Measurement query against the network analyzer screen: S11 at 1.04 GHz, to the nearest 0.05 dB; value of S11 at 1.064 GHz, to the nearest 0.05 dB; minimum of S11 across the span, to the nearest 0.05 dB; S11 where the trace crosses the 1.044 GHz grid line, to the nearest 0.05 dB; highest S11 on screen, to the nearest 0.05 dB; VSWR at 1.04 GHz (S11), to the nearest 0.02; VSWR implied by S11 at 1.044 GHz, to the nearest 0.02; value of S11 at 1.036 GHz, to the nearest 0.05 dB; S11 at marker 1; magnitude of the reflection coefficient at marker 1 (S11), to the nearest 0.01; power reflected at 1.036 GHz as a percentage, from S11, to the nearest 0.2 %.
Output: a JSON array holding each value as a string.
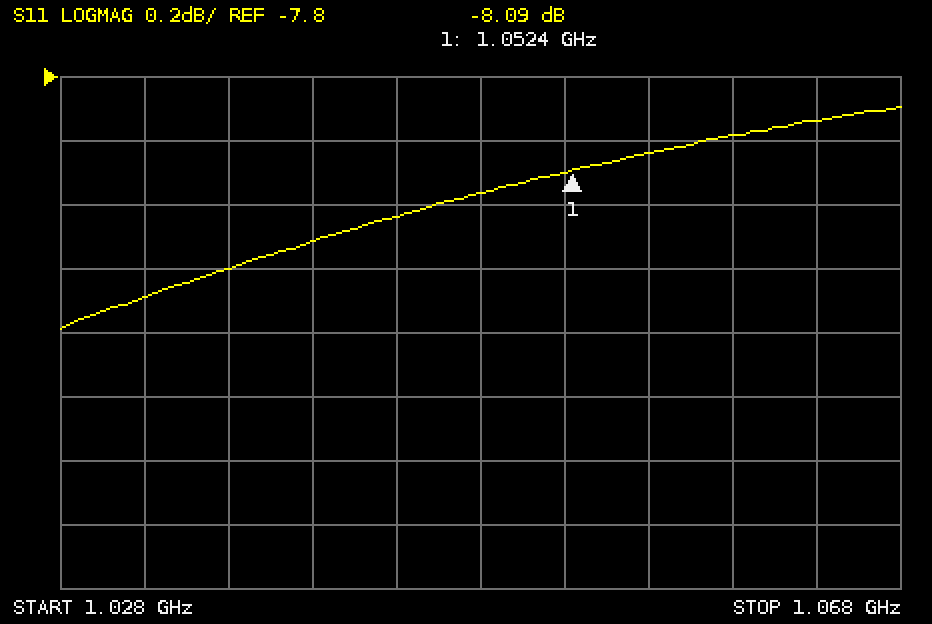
["-8.30 dB", "-7.95 dB", "-8.60 dB", "-8.25 dB", "-7.90 dB", "2.24", "2.26", "-8.40 dB", "-8.09 dB", "0.39", "14.4 %"]
